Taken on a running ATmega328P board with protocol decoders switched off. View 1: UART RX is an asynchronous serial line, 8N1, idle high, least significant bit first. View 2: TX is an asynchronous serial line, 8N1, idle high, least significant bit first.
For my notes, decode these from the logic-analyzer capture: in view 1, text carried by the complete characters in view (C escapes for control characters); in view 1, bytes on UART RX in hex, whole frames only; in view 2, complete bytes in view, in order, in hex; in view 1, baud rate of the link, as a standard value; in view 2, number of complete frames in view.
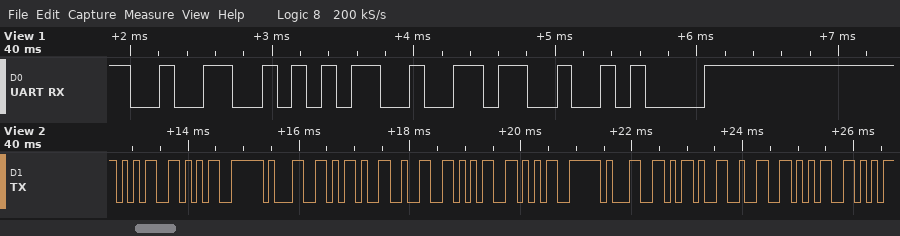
"256\n"
0x32 0x35 0x36 0x0A
0x35 0x35 0x31 0x2D 0x32 0x35 0x35 0x31 0x2D 0x32 0x35
9600 baud
11
